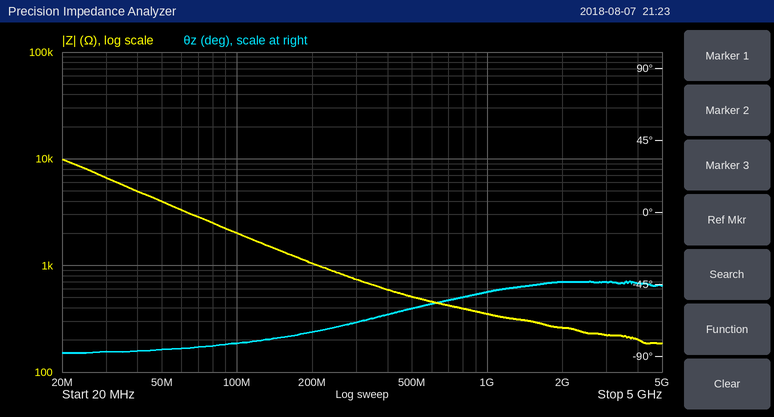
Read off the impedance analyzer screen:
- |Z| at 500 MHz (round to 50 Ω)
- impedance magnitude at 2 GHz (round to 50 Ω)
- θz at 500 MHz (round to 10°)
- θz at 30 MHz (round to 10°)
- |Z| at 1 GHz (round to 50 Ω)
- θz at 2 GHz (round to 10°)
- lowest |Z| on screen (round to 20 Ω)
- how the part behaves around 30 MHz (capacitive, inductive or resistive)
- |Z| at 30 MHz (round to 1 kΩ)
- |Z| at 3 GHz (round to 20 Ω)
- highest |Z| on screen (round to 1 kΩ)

500 Ω
250 Ω
-60°
-90°
350 Ω
-40°
180 Ω
capacitive
7 kΩ
220 Ω
10 kΩ
